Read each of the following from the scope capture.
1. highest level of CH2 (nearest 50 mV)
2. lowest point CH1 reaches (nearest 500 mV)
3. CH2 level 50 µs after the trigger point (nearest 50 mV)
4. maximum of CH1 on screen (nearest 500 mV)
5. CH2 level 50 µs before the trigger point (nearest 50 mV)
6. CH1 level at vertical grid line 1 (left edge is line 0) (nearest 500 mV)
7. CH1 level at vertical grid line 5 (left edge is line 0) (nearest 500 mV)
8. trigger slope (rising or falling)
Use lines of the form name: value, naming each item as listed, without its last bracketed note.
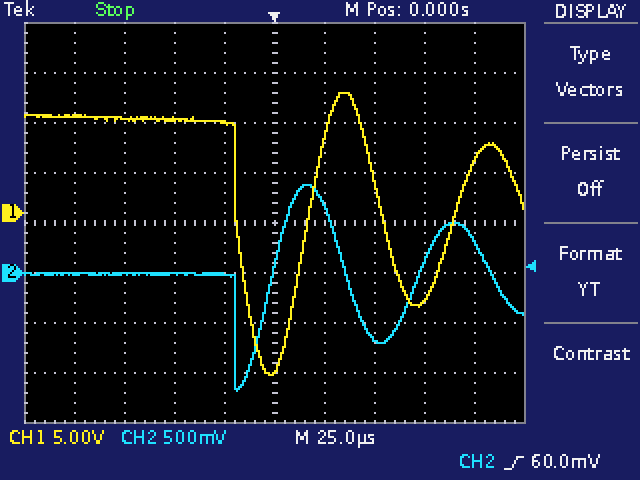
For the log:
highest level of CH2: 900 mV
lowest point CH1 reaches: -16.0 V
CH2 level 50 µs after the trigger point: -650 mV
maximum of CH1 on screen: 12.0 V
CH2 level 50 µs before the trigger point: 0 mV
CH1 level at vertical grid line 1 (left edge is line 0): 9.5 V
CH1 level at vertical grid line 5 (left edge is line 0): -15.5 V
trigger slope: rising
